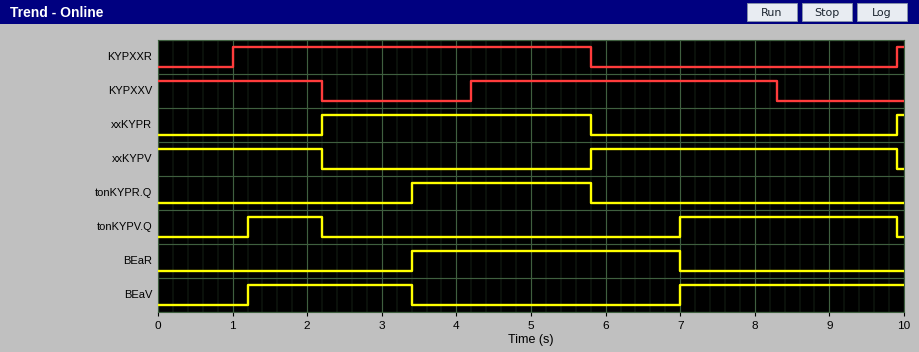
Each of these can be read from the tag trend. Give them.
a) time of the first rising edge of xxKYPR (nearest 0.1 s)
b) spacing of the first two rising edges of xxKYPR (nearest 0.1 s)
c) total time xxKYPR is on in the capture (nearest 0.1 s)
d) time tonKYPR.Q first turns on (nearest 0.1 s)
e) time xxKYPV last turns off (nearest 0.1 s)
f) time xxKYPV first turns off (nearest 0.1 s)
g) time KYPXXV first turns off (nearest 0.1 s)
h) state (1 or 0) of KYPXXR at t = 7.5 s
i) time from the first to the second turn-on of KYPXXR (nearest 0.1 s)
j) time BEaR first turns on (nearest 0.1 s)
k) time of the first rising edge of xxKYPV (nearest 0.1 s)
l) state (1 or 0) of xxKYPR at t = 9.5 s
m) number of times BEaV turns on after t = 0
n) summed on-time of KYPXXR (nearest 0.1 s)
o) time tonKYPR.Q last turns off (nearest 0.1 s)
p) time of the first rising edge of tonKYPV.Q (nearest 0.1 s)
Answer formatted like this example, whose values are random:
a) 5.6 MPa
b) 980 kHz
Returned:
a) 2.2 s
b) 7.7 s
c) 3.7 s
d) 3.4 s
e) 9.9 s
f) 2.2 s
g) 2.2 s
h) 0
i) 8.9 s
j) 3.4 s
k) 5.8 s
l) 0
m) 2
n) 4.9 s
o) 5.8 s
p) 1.2 s
